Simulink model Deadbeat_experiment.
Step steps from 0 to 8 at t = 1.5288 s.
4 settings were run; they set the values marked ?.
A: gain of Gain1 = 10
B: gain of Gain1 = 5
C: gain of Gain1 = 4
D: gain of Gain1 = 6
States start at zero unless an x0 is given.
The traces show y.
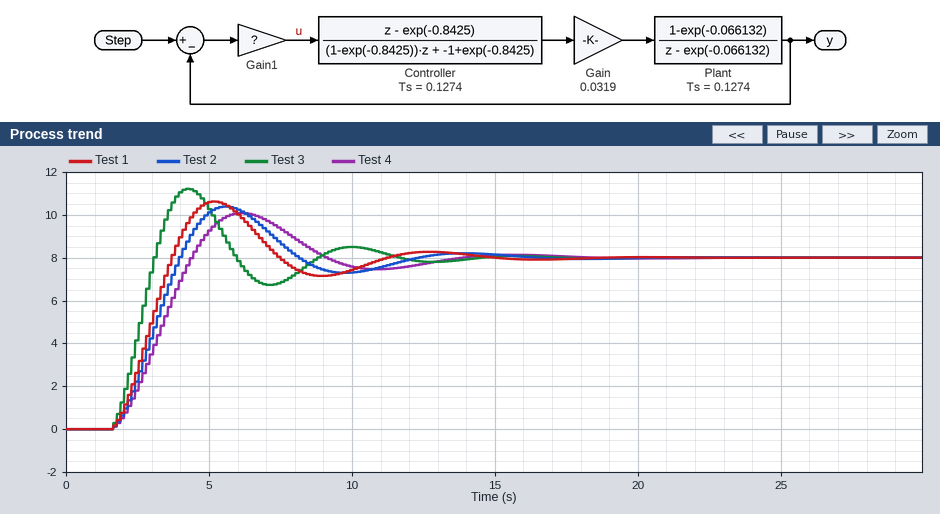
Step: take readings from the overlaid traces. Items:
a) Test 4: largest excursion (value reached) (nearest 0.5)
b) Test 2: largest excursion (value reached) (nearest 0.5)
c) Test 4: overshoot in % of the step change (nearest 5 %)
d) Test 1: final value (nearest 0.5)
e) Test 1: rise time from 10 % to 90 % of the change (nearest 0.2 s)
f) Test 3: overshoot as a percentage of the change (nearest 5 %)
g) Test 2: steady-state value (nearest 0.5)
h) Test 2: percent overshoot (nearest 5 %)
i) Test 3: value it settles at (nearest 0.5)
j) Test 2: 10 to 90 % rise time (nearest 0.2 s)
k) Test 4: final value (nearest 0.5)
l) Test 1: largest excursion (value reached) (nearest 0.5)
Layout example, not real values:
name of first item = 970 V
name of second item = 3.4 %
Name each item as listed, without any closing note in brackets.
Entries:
Test 4: largest excursion (value reached) = 10.0
Test 2: largest excursion (value reached) = 10.5
Test 4: overshoot in % of the step change = 25 %
Test 1: final value = 8.0
Test 1: rise time from 10 % to 90 % of the change = 1.6 s
Test 3: overshoot as a percentage of the change = 40 %
Test 2: steady-state value = 8.0
Test 2: percent overshoot = 30 %
Test 3: value it settles at = 8.0
Test 2: 10 to 90 % rise time = 1.6 s
Test 4: final value = 8.0
Test 1: largest excursion (value reached) = 10.5
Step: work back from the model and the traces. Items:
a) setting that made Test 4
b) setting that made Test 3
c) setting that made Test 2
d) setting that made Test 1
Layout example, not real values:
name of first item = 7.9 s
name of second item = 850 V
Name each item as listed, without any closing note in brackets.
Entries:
setting that made Test 4 = C
setting that made Test 3 = A
setting that made Test 2 = B
setting that made Test 1 = D
